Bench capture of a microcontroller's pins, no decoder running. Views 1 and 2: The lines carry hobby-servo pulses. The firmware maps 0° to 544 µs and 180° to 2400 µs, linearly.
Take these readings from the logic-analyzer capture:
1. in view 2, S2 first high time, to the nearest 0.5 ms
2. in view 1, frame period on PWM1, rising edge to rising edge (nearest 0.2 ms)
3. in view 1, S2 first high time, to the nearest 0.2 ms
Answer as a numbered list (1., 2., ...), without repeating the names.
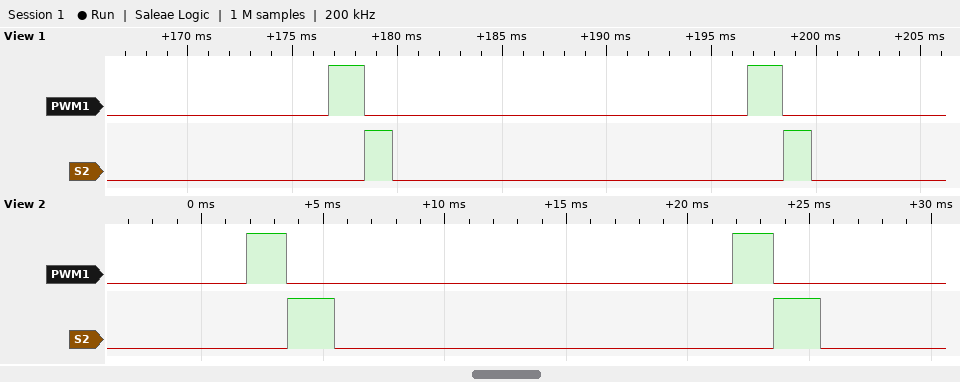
1. 2.0 ms
2. 20.0 ms
3. 1.4 ms
